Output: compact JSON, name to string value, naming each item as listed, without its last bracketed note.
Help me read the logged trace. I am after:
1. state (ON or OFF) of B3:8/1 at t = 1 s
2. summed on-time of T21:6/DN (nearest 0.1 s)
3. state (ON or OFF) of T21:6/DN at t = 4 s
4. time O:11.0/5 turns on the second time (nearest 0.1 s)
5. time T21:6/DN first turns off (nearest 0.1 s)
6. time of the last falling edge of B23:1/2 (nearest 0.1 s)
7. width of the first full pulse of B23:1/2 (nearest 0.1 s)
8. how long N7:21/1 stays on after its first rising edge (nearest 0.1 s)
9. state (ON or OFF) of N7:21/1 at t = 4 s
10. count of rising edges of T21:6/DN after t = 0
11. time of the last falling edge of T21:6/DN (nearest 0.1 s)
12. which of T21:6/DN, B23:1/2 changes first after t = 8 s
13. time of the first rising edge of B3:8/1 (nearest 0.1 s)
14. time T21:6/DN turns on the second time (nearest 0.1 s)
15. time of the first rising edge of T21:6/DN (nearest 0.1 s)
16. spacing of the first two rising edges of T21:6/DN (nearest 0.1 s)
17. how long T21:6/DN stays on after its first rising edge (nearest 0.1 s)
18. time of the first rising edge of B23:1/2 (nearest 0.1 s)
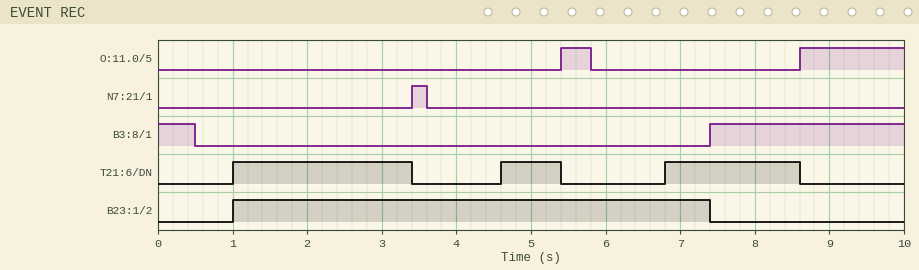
{"state (ON or OFF) of B3:8/1 at t = 1 s": "OFF", "summed on-time of T21:6/DN": "5.0 s", "state (ON or OFF) of T21:6/DN at t = 4 s": "OFF", "time O:11.0/5 turns on the second time": "8.6 s", "time T21:6/DN first turns off": "3.4 s", "time of the last falling edge of B23:1/2": "7.4 s", "width of the first full pulse of B23:1/2": "6.4 s", "how long N7:21/1 stays on after its first rising edge": "0.2 s", "state (ON or OFF) of N7:21/1 at t = 4 s": "OFF", "count of rising edges of T21:6/DN after t = 0": "3", "time of the last falling edge of T21:6/DN": "8.6 s", "which of T21:6/DN, B23:1/2 changes first after t = 8 s": "T21:6/DN", "time of the first rising edge of B3:8/1": "7.4 s", "time T21:6/DN turns on the second time": "4.6 s", "time of the first rising edge of T21:6/DN": "1.0 s", "spacing of the first two rising edges of T21:6/DN": "3.6 s", "how long T21:6/DN stays on after its first rising edge": "2.4 s", "time of the first rising edge of B23:1/2": "1.0 s"}
